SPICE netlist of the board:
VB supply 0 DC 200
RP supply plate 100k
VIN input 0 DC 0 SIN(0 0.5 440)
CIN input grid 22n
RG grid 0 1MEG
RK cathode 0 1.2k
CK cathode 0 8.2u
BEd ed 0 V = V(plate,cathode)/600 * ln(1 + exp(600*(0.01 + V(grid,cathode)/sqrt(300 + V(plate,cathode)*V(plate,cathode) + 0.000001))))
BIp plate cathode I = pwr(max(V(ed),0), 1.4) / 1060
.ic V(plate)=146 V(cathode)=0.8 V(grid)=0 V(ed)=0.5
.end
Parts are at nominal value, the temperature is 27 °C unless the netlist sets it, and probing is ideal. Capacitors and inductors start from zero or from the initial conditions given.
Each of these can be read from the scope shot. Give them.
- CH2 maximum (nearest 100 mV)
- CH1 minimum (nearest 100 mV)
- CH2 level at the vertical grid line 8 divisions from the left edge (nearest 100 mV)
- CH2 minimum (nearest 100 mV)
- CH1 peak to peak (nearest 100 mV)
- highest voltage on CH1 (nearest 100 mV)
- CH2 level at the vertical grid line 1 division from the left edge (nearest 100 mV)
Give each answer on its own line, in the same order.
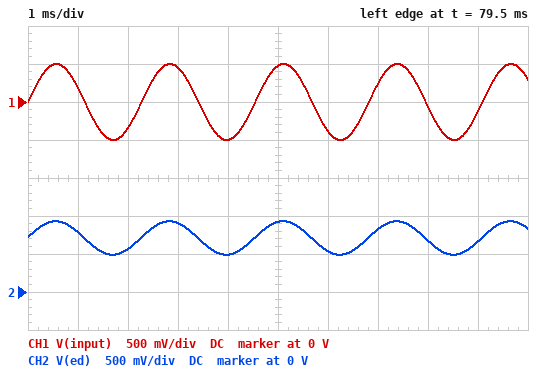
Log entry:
900 mV
-500 mV
700 mV
500 mV
1.0 V
500 mV
800 mV
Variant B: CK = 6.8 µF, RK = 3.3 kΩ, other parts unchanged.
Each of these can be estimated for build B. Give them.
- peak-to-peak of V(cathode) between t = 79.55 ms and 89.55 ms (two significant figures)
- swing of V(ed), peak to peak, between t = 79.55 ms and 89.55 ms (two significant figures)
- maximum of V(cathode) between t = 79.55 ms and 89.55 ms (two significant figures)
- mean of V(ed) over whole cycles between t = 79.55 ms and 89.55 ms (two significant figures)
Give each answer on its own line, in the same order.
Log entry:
23 mV
430 mV
1.2 V
500 mV
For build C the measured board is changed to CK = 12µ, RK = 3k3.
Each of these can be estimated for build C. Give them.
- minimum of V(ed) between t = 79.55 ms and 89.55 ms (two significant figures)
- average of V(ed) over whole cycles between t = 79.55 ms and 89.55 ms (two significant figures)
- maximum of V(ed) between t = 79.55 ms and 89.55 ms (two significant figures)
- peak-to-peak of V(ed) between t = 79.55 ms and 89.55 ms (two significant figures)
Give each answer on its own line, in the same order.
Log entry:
290 mV
500 mV
720 mV
430 mV
